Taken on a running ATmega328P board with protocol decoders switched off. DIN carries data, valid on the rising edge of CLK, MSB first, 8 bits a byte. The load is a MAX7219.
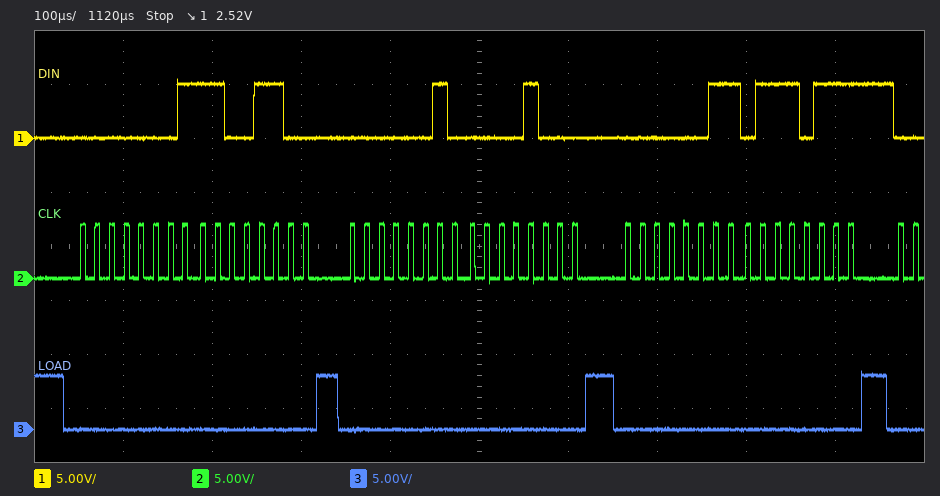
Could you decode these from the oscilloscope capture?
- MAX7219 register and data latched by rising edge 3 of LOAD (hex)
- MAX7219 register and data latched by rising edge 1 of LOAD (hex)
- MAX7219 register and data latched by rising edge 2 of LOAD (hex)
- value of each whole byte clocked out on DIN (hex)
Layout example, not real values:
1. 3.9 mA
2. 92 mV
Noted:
1. register 0x3, data 0x77
2. register 0x1, data 0xCC
3. register 0x2, data 0x08
4. 0x01 0xCC 0x02 0x08 0x03 0x77
